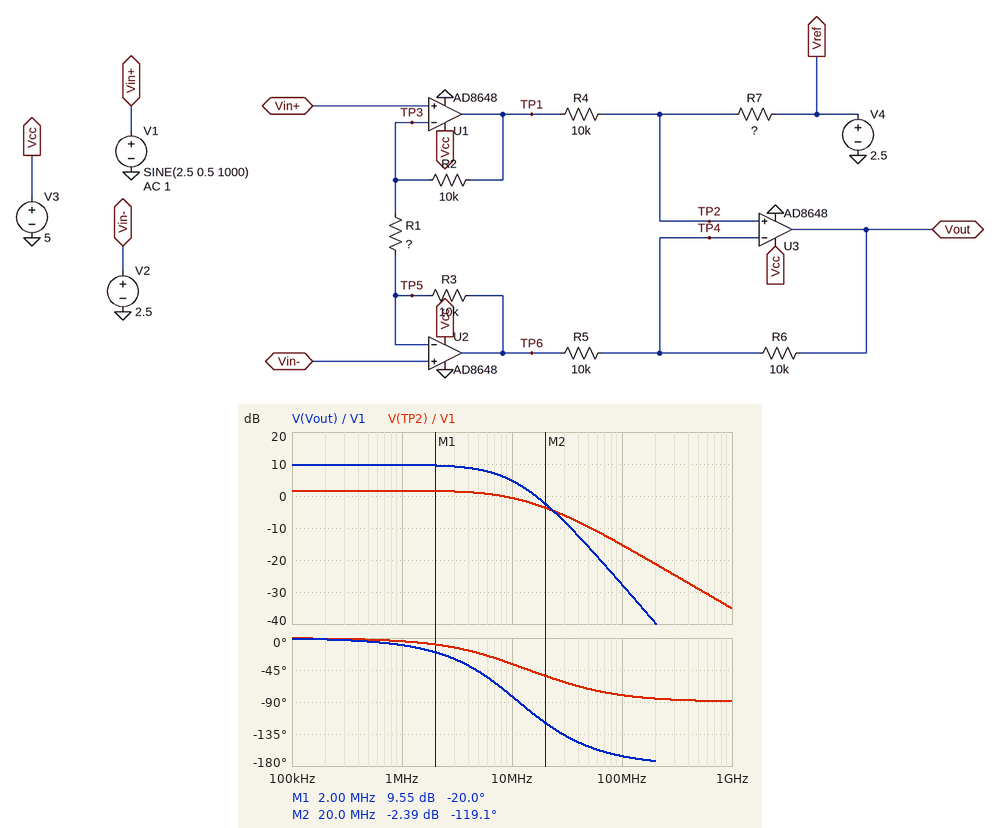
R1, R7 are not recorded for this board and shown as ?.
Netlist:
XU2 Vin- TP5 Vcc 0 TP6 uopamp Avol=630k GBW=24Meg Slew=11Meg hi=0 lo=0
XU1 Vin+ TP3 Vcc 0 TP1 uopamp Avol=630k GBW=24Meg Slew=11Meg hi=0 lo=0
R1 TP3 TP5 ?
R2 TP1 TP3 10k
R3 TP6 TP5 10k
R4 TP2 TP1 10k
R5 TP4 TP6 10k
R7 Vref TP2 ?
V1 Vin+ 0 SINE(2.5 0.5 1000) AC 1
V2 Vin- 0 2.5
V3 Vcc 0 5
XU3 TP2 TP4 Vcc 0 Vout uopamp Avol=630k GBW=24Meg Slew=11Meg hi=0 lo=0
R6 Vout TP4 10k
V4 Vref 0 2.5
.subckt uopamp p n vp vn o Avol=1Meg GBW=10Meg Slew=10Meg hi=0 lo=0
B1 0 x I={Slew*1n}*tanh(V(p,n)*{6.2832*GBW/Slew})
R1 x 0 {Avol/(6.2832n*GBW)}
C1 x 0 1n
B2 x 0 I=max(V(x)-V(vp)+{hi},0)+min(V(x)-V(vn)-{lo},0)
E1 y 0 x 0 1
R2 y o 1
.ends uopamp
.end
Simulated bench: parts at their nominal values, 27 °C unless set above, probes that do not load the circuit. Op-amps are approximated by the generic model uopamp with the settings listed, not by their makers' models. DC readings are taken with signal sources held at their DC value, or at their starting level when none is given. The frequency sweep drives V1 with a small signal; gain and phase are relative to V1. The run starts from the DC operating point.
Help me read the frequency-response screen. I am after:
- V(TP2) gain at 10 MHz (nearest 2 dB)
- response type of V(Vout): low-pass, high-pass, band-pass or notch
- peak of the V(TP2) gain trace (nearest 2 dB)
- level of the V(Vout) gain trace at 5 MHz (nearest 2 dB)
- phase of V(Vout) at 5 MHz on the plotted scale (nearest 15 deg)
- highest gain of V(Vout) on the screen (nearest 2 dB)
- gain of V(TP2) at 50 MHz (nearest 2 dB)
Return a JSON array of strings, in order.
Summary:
["0 dB", "low-pass", "2 dB", "8 dB", "-45 deg", "10 dB", "-10 dB"]
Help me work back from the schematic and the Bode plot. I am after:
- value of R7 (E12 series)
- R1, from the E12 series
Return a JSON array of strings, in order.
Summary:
["27 kΩ", "15 kΩ"]
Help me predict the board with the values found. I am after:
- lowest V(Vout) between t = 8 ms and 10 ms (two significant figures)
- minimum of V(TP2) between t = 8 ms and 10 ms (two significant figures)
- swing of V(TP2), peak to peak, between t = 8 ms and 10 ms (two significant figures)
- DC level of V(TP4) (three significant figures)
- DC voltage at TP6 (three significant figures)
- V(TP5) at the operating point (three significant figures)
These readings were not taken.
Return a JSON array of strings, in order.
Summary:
["950 mV", "1.9 V", "1.2 V", "2.50 V", "2.50 V", "2.50 V"]
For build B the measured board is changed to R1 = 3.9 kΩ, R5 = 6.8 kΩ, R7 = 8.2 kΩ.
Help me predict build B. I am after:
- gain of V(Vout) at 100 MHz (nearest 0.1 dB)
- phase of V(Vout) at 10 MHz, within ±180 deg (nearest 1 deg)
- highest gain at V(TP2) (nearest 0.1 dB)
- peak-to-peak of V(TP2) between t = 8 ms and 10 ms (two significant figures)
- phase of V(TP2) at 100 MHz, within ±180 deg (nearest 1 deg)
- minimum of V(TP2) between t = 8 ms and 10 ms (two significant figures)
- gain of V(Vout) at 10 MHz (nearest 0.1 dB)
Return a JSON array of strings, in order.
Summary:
["-31.7 dB", "-117 deg", "4.1 dB", "1.6 V", "-82 deg", "1.7 V", "5.7 dB"]
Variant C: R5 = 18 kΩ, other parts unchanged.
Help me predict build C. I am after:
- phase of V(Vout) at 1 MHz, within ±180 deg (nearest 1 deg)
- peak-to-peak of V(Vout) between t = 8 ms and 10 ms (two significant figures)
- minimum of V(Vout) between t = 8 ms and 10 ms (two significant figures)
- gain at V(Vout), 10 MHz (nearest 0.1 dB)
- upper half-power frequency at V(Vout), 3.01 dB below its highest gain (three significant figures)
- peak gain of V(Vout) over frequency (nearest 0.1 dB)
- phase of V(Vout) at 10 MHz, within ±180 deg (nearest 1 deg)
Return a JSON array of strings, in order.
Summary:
["-9 deg", "2.3 V", "1.4 V", "2.9 dB", "8.13 MHz", "7.1 dB", "-74 deg"]
